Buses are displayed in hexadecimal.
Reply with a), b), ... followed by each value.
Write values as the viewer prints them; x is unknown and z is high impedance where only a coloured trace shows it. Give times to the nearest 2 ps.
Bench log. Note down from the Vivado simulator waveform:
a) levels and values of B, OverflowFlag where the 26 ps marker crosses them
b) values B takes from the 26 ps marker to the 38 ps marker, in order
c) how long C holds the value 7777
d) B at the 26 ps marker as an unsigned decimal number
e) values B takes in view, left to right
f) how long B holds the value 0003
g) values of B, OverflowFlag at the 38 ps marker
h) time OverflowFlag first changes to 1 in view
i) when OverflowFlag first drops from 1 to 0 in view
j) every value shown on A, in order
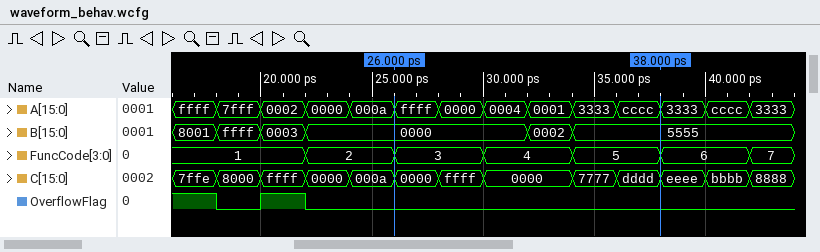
a) B=0000, OverflowFlag=0
b) 0000, 0002, 5555
c) 2 ps
d) 0
e) 8001, ffff, 0003, 0000, 0002, 5555
f) 2 ps
g) B=5555, OverflowFlag=0
h) 20 ps
i) 18 ps
j) ffff, 7fff, 0002, 0000, 000a, ffff, 0000, 0004, 0001, 3333, cccc, 3333, cccc, 3333
